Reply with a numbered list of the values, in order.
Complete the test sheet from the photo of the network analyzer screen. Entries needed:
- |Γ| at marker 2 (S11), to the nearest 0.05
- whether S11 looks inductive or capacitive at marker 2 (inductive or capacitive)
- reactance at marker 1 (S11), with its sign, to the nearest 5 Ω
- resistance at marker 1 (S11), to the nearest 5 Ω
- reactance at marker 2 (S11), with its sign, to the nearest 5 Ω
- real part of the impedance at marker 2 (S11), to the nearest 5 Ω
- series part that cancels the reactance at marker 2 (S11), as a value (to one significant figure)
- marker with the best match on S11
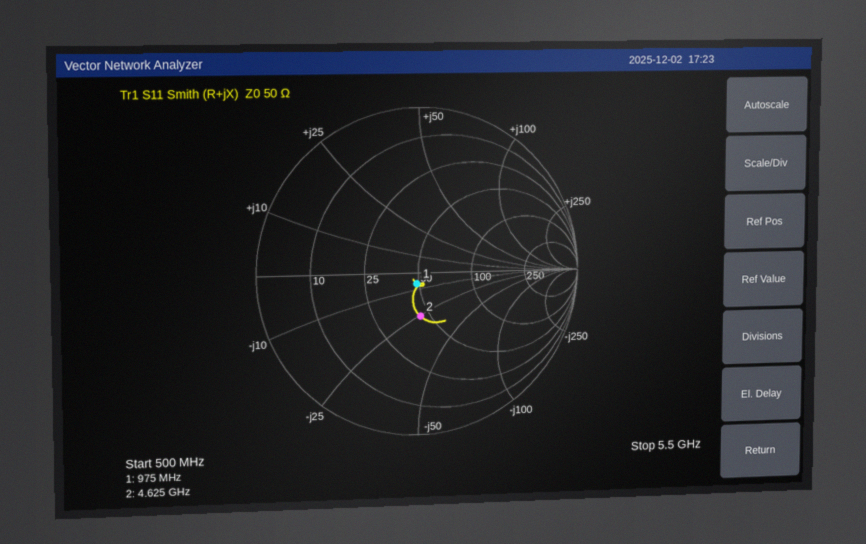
1. 0.25
2. capacitive
3. -5 Ω
4. 50 Ω
5. -25 Ω
6. 45 Ω
7. 900 pH
8. marker 1
